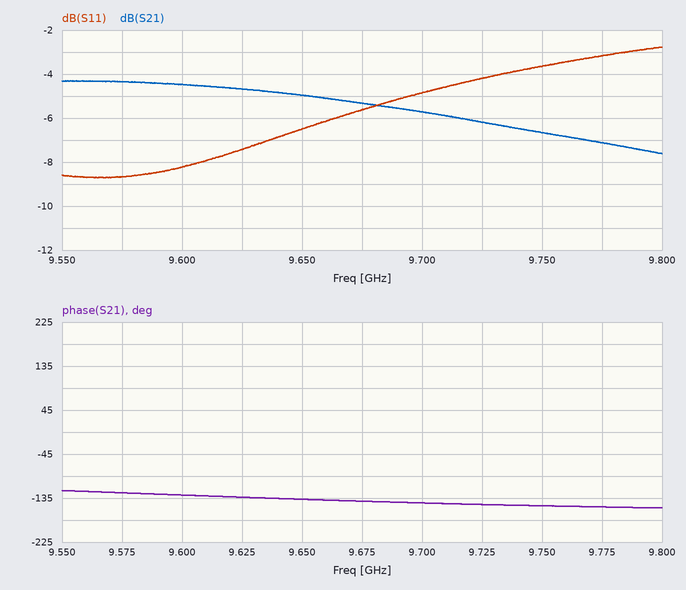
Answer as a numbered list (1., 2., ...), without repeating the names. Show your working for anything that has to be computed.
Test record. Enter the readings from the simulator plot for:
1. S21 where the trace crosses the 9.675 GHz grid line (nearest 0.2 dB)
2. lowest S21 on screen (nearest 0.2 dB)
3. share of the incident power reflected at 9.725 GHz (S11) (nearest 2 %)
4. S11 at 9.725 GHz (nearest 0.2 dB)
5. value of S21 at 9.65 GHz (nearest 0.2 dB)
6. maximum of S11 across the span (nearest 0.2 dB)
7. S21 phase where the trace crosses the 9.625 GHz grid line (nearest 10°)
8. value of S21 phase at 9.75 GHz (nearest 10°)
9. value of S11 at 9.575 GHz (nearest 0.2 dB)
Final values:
1. -5.4 dB
2. -7.6 dB
3. 10^(-4.2/10) ≈ 38 %
4. -4.2 dB
5. -5.0 dB
6. -2.8 dB
7. -130°
8. -150°
9. -8.6 dB
